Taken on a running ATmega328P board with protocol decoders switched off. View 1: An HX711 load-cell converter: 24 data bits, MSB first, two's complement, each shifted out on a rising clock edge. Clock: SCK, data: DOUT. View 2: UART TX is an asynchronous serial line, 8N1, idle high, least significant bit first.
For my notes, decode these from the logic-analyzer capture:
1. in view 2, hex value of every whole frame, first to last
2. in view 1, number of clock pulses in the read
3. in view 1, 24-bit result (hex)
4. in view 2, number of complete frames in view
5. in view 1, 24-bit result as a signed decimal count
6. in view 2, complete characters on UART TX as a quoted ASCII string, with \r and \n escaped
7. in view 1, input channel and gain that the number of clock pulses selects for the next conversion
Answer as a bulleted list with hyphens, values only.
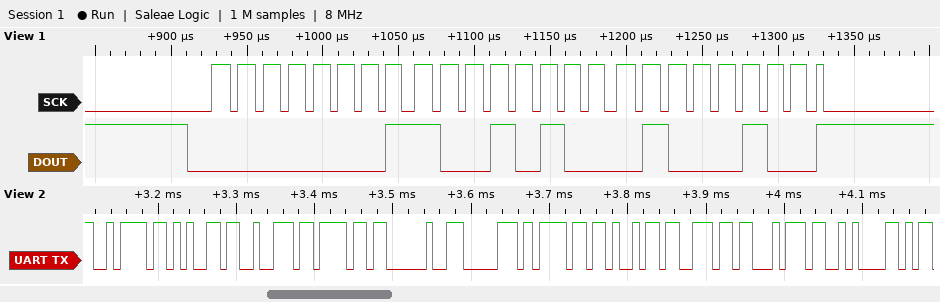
- 7A 65 72 6F 20 70 6F 69 6E 74 0A
- 25
- 0x019444
- 11
- 103492
- "zero point\n"
- channel A, gain 128
